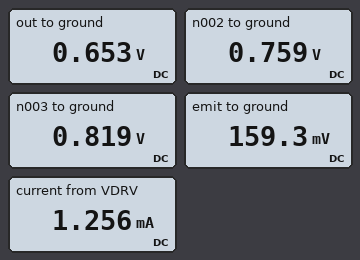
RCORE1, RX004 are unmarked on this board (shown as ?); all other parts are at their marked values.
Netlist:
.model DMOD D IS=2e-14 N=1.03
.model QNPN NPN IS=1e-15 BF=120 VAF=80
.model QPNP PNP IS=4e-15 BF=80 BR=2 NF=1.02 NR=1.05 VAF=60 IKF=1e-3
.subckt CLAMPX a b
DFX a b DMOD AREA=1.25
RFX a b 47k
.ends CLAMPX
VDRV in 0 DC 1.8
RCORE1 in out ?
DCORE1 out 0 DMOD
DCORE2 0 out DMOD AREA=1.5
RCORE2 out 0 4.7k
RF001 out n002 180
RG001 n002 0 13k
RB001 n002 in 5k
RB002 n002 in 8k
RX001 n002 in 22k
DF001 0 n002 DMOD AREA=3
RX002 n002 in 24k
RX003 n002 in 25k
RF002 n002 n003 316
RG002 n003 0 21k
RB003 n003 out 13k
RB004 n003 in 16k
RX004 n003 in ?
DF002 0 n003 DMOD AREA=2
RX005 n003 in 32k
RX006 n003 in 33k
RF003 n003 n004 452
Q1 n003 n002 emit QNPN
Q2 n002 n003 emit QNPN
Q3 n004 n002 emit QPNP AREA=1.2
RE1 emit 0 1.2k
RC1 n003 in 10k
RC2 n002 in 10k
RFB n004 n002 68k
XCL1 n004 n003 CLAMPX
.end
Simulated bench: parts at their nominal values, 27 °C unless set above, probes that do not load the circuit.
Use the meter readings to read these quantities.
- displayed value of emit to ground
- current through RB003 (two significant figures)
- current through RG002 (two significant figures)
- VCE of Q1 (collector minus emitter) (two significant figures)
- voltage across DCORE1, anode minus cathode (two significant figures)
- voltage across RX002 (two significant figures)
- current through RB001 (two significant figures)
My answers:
159.3 mV
13 µA
39 µA
660 mV
650 mV
1.0 V
210 µA
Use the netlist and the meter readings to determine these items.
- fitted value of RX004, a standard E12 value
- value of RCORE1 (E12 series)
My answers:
27 kΩ
2.7 kΩ
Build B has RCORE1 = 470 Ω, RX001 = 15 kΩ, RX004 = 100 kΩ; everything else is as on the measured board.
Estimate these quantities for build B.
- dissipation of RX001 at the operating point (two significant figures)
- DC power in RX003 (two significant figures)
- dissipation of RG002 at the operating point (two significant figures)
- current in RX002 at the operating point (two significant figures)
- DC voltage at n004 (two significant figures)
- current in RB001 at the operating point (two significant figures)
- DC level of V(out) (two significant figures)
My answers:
69 µW
41 µW
33 µW
42 µA
830 mV
200 µA
680 mV
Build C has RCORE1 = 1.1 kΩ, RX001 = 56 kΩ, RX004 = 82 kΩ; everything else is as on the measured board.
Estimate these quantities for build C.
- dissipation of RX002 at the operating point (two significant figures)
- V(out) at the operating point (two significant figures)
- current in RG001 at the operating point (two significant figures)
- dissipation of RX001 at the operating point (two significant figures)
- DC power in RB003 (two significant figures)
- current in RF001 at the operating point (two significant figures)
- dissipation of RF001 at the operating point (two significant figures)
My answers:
45 µW
670 mV
59 µA
19 µW
1.7 µW
540 µA
52 µW
